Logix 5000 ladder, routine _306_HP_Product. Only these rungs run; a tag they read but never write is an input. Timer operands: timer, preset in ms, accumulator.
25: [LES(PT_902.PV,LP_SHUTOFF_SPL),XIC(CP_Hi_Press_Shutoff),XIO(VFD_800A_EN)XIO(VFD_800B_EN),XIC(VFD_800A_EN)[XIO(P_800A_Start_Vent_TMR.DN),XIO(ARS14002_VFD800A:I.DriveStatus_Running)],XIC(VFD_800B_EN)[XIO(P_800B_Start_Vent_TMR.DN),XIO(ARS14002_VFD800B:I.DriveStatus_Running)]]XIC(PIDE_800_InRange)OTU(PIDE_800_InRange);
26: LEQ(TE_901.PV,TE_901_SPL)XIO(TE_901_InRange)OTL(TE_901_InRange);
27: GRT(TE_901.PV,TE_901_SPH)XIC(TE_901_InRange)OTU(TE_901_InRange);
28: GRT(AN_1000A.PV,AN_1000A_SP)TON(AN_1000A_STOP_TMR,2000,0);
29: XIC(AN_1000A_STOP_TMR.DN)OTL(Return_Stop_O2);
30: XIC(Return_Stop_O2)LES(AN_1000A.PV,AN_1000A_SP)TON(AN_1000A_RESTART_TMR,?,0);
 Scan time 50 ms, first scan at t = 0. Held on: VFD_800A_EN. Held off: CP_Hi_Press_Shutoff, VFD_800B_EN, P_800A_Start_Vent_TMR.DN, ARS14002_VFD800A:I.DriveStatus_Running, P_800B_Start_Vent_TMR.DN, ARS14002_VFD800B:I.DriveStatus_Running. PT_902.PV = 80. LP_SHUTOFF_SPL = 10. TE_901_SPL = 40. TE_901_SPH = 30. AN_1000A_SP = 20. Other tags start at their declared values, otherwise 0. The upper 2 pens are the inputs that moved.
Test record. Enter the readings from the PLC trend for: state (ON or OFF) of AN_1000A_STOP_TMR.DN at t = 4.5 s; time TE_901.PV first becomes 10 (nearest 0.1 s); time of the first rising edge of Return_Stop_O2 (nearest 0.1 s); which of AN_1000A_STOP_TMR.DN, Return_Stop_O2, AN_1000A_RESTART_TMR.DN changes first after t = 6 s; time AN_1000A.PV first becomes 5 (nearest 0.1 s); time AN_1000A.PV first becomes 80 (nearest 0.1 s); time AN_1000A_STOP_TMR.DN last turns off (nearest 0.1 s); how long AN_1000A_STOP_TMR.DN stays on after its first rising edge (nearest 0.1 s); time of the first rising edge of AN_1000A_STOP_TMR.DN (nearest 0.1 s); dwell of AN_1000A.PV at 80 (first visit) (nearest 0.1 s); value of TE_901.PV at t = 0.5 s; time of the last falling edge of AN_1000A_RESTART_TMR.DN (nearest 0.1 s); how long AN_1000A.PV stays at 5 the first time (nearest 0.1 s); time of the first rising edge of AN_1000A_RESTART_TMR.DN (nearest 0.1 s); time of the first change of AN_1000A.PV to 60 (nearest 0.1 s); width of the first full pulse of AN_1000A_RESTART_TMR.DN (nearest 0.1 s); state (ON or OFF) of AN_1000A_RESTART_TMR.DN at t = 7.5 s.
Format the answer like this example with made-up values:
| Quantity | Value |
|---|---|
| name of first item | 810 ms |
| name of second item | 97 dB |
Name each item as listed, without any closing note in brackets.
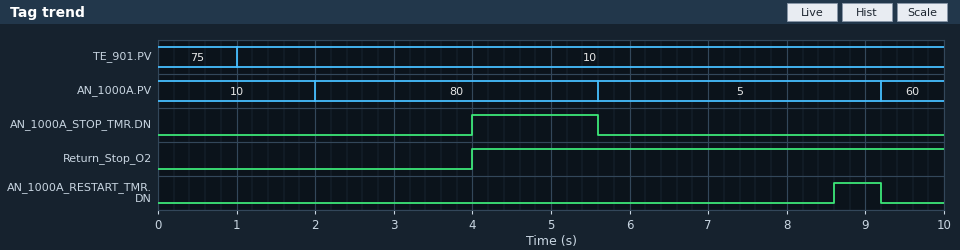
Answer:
| Quantity | Value |
|---|---|
| state (ON or OFF) of AN_1000A_STOP_TMR.DN at t = 4.5 s | ON |
| time TE_901.PV first becomes 10 | 1.0 s |
| time of the first rising edge of Return_Stop_O2 | 4.0 s |
| which of AN_1000A_STOP_TMR.DN, Return_Stop_O2, AN_1000A_RESTART_TMR.DN changes first after t = 6 s | AN_1000A_RESTART_TMR.DN |
| time AN_1000A.PV first becomes 5 | 5.6 s |
| time AN_1000A.PV first becomes 80 | 2.0 s |
| time AN_1000A_STOP_TMR.DN last turns off | 5.6 s |
| how long AN_1000A_STOP_TMR.DN stays on after its first rising edge | 1.6 s |
| time of the first rising edge of AN_1000A_STOP_TMR.DN | 4.0 s |
| dwell of AN_1000A.PV at 80 (first visit) | 3.6 s |
| value of TE_901.PV at t = 0.5 s | 75 |
| time of the last falling edge of AN_1000A_RESTART_TMR.DN | 9.2 s |
| how long AN_1000A.PV stays at 5 the first time | 3.6 s |
| time of the first rising edge of AN_1000A_RESTART_TMR.DN | 8.6 s |
| time of the first change of AN_1000A.PV to 60 | 9.2 s |
| width of the first full pulse of AN_1000A_RESTART_TMR.DN | 0.6 s |
| state (ON or OFF) of AN_1000A_RESTART_TMR.DN at t = 7.5 s | OFF |
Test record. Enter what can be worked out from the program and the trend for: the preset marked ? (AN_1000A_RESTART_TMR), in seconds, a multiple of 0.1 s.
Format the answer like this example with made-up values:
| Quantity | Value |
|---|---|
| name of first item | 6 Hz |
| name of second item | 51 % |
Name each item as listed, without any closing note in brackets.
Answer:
| Quantity | Value |
|---|---|
| the preset marked ? (AN_1000A_RESTART_TMR), in seconds, a multiple of 0.1 s | 3.0 s |
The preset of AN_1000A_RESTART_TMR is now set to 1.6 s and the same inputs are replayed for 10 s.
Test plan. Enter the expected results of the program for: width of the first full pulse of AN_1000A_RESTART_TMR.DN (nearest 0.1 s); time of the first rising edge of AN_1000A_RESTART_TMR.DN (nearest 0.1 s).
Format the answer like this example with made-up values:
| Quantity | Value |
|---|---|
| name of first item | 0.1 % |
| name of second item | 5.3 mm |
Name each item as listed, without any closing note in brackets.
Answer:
| Quantity | Value |
|---|---|
| width of the first full pulse of AN_1000A_RESTART_TMR.DN | 2.0 s |
| time of the first rising edge of AN_1000A_RESTART_TMR.DN | 7.2 s |
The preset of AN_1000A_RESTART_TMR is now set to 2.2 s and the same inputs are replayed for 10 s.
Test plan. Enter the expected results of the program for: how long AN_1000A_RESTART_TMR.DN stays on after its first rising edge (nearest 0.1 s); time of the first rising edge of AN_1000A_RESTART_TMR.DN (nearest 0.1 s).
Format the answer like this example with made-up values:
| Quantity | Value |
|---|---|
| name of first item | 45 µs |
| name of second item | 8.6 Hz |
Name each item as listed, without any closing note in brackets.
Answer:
| Quantity | Value |
|---|---|
| how long AN_1000A_RESTART_TMR.DN stays on after its first rising edge | 1.4 s |
| time of the first rising edge of AN_1000A_RESTART_TMR.DN | 7.8 s |
